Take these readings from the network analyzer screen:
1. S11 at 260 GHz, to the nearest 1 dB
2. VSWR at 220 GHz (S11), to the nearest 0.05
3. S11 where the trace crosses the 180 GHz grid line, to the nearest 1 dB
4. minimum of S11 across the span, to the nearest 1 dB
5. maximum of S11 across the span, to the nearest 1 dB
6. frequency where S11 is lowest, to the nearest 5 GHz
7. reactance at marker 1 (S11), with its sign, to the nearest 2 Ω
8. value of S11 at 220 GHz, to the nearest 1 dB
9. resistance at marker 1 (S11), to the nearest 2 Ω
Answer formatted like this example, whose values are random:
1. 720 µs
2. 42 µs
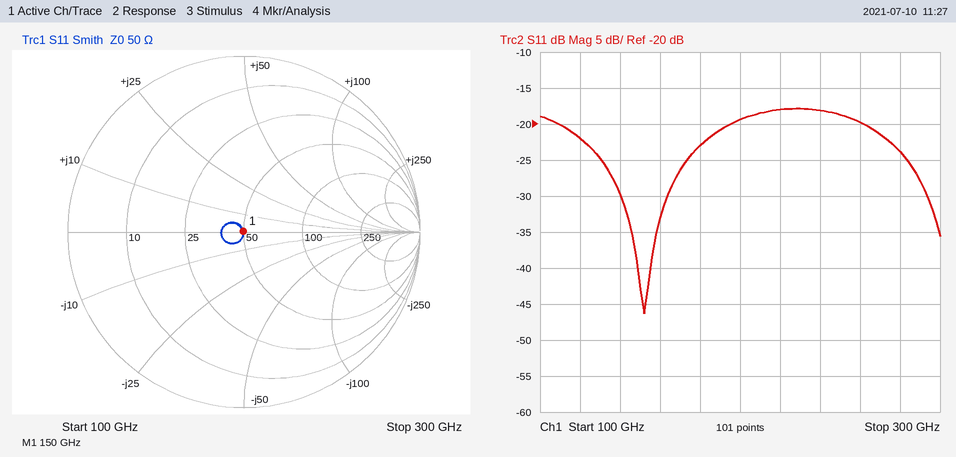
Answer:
1. -20 dB
2. 1.30
3. -23 dB
4. -46 dB
5. -18 dB
6. 150 GHz
7. 0 Ω
8. -18 dB
9. 50 Ω
